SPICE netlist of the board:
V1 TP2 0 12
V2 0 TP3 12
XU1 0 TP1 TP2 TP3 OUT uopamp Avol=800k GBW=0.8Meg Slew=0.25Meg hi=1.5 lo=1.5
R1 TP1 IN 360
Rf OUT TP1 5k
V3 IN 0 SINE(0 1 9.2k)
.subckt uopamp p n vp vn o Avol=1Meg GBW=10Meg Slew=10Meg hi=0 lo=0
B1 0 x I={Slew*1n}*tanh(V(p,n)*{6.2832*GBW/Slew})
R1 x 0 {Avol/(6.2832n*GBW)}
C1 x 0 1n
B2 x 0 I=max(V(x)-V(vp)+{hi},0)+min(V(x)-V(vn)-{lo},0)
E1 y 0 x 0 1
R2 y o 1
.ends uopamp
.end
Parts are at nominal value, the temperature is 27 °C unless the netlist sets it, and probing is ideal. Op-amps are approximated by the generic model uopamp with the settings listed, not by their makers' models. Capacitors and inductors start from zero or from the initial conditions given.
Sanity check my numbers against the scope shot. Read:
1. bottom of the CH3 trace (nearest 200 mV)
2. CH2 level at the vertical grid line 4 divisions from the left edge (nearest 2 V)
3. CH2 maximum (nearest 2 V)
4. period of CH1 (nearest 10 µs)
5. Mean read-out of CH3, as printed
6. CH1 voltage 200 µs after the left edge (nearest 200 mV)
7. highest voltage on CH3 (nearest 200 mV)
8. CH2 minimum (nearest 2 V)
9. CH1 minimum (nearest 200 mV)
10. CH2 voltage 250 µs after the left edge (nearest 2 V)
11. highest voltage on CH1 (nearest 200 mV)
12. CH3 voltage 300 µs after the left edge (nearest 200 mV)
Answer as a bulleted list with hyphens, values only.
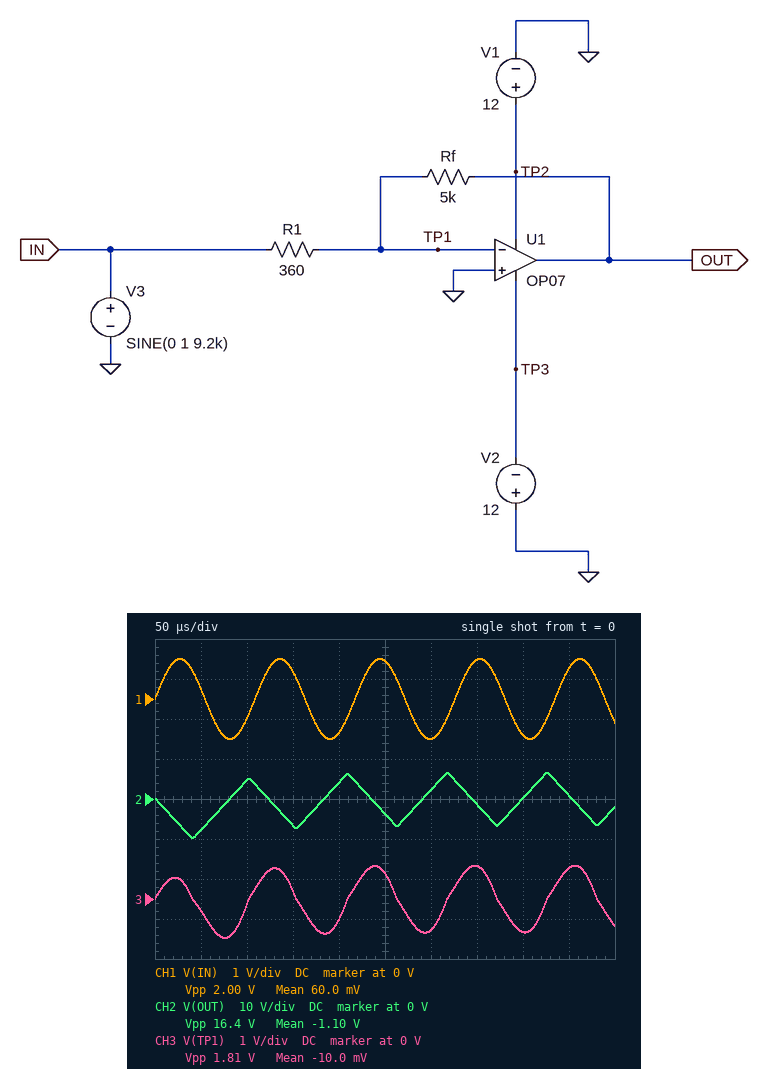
- -1.0 V
- 4 V
- 6 V
- 110 µs
- -10.0 mV
- -800 mV
- 800 mV
- -10 V
- -1.0 V
- -4 V
- 1.0 V
- -800 mV
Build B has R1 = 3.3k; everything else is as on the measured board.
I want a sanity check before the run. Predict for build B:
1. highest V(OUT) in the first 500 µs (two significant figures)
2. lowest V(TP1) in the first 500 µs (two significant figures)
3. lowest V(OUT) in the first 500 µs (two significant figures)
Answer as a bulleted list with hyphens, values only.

- 1.5 V
- -18 mV
- -1.5 V
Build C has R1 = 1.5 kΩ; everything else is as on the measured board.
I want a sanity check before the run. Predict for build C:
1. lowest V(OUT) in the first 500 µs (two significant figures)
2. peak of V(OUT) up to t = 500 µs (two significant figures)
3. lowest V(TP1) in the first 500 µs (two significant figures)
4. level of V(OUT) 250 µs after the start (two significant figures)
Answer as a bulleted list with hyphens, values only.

- -3.3 V
- 3.3 V
- -50 mV
- -3.2 V
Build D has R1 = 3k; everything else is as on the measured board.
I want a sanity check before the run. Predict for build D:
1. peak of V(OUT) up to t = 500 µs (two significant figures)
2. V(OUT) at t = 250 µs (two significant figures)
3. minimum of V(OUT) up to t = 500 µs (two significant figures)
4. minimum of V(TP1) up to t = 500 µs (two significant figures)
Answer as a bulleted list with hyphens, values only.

- 1.7 V
- -1.6 V
- -1.7 V
- -20 mV
